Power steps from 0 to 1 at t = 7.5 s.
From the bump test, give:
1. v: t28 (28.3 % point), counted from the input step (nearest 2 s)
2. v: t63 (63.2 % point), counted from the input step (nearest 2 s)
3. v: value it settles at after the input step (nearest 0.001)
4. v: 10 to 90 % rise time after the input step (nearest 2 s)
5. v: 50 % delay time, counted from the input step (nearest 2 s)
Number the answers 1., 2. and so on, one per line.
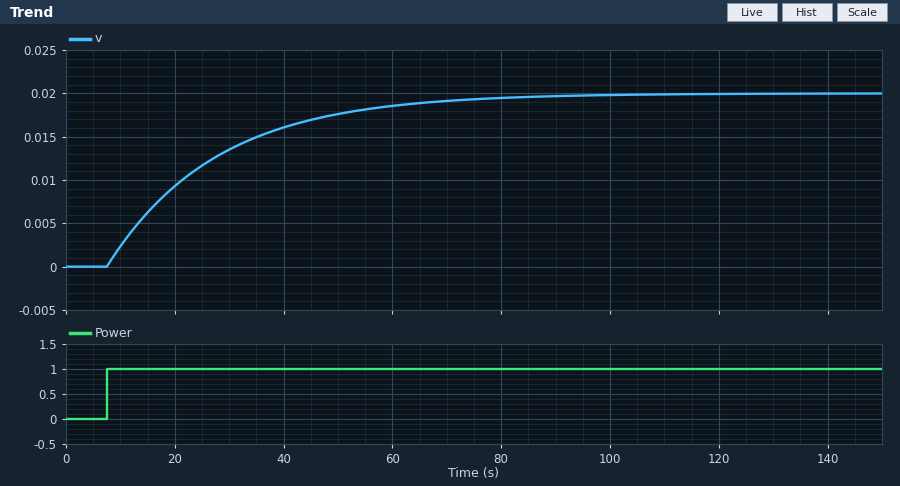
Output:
1. 6 s
2. 20 s
3. 0.020
4. 44 s
5. 14 s
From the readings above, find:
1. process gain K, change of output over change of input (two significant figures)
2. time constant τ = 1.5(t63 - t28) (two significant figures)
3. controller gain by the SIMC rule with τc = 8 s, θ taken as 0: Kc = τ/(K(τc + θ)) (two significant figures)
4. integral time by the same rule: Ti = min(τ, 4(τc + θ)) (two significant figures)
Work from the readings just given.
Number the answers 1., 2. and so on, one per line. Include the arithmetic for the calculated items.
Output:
1. (0.02 - 0) / 1 = 0.020
2. 1.5 × (20 - 6) = 21 s
3. 21 / (0.02 × (8 + 0)) = 130
4. min(21, 4 × (8 + 0)) = 21 s
